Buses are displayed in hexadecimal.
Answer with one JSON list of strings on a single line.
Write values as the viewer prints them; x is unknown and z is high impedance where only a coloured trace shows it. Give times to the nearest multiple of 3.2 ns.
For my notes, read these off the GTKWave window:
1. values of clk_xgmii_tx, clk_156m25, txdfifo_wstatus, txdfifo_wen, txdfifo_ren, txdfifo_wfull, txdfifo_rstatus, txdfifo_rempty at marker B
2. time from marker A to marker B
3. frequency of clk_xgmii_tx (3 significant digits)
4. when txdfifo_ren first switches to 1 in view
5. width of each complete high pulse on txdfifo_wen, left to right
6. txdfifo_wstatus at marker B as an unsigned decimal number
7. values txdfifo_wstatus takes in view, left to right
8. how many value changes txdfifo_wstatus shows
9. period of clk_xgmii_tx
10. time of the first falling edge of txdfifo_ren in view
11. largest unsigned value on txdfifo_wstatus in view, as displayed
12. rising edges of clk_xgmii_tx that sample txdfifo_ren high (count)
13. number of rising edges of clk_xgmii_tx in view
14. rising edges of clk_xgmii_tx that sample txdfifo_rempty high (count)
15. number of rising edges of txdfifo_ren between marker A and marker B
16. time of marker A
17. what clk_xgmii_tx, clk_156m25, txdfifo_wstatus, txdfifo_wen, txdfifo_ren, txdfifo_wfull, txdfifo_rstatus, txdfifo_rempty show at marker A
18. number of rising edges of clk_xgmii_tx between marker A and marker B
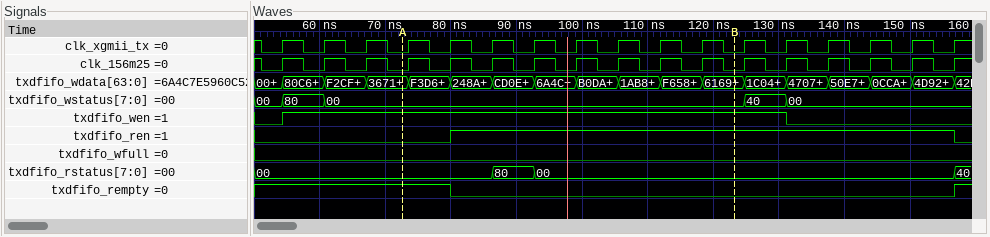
["clk_xgmii_tx=0, clk_156m25=0, txdfifo_wstatus=00, txdfifo_wen=1, txdfifo_ren=1, txdfifo_wfull=0, txdfifo_rstatus=00, txdfifo_rempty=0", "51.2 ns", "156 MHz", "80 ns", "76.8 ns", "0", "00, 80, 00, 40, 00", "4", "6.4 ns", "156.8 ns", "80", "12", "17", "5", "1", "73.6 ns", "clk_xgmii_tx=0, clk_156m25=0, txdfifo_wstatus=00, txdfifo_wen=1, txdfifo_ren=0, txdfifo_wfull=0, txdfifo_rstatus=00, txdfifo_rempty=1", "8"]
